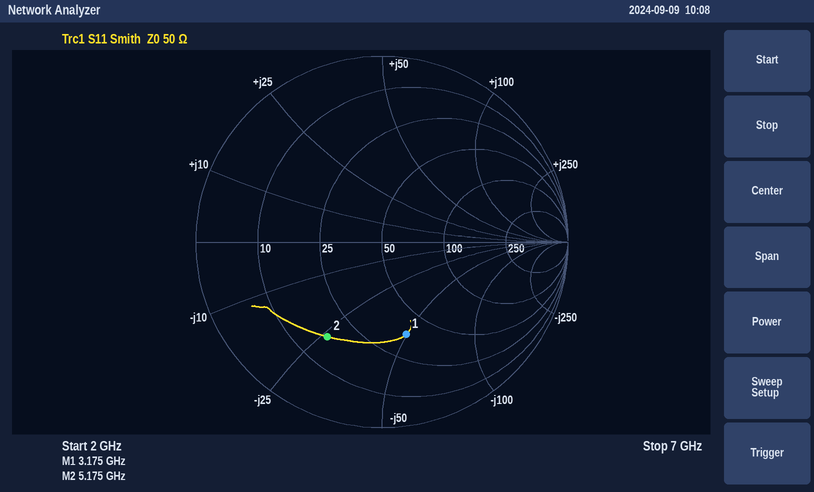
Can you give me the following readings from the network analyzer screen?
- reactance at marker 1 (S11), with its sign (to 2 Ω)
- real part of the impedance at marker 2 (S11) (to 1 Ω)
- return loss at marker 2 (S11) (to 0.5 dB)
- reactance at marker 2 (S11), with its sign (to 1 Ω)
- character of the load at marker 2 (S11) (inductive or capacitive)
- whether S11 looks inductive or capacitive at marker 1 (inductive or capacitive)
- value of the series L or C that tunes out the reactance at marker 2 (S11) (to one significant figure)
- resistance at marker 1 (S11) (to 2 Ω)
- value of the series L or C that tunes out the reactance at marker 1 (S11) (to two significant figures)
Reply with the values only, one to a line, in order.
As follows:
-50 Ω
17 Ω
4.5 dB
-26 Ω
capacitive
capacitive
800 pH
36 Ω
2.5 nH
